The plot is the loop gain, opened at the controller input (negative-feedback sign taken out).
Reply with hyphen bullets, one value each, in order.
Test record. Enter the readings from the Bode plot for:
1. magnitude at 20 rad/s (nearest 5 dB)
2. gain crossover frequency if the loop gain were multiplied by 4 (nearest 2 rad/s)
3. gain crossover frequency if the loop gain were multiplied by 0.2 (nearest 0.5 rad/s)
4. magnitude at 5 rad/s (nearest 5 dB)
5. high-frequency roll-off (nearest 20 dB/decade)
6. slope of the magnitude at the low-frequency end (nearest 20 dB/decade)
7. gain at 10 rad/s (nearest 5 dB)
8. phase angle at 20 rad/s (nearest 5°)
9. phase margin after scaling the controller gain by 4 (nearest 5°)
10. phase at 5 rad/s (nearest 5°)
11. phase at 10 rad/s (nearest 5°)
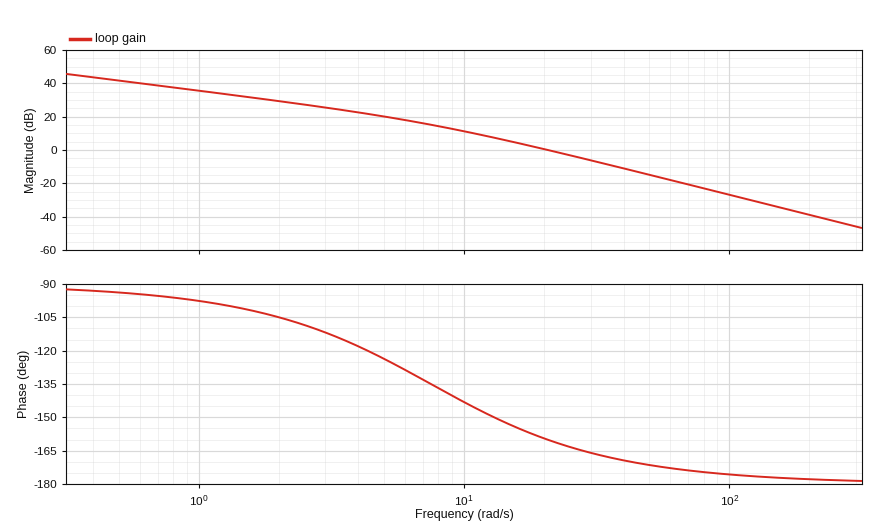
- 0 dB
- 42 rad/s
- 8.0 rad/s
- 20 dB
- -40 dB/decade
- -20 dB/decade
- 10 dB
- -160°
- 10°
- -125°
- -145°
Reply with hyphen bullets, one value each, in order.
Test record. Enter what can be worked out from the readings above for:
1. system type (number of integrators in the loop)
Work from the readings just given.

- 1
